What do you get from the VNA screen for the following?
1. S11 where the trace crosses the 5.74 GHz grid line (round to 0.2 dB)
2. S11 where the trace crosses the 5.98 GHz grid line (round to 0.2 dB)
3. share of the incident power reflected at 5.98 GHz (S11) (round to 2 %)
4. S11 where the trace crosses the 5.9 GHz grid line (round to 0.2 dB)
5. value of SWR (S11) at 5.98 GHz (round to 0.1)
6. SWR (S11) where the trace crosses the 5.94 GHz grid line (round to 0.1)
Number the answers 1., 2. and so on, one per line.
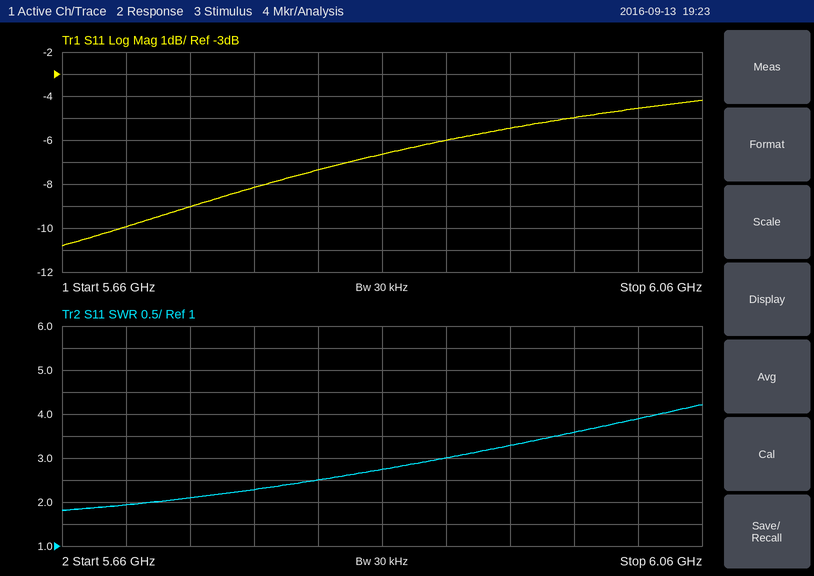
1. -9.0 dB
2. -5.0 dB
3. 32 %
4. -6.0 dB
5. 3.6
6. 3.3
